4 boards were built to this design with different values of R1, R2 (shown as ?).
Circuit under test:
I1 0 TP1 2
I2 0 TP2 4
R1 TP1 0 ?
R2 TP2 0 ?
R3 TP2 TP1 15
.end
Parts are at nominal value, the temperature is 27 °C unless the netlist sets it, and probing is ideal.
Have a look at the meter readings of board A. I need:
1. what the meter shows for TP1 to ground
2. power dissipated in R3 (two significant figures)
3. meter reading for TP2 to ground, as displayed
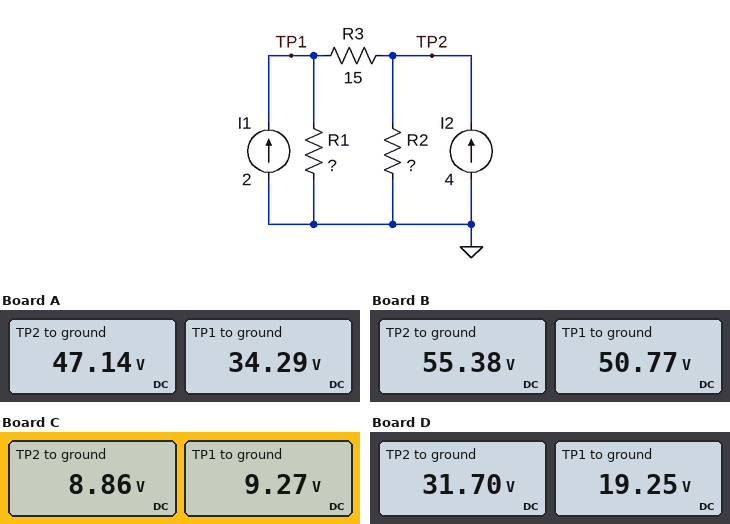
34.29 V
11 W
47.14 V
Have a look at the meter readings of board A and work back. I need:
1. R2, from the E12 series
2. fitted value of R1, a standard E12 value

15 Ω
12 Ω
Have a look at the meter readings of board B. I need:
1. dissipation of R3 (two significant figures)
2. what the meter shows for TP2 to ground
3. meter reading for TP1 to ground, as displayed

1.4 W
55.38 V
50.77 V
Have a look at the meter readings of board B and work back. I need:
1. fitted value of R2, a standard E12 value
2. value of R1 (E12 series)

15 Ω
22 Ω
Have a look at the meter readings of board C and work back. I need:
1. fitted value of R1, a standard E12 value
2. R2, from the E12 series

4.7 Ω
2.2 Ω
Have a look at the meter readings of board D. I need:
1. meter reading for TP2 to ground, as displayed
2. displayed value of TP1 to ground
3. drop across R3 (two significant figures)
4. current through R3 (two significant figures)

31.70 V
19.25 V
12 V
830 mA
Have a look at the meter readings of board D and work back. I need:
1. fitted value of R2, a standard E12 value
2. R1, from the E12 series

10 Ω
6.8 Ω
